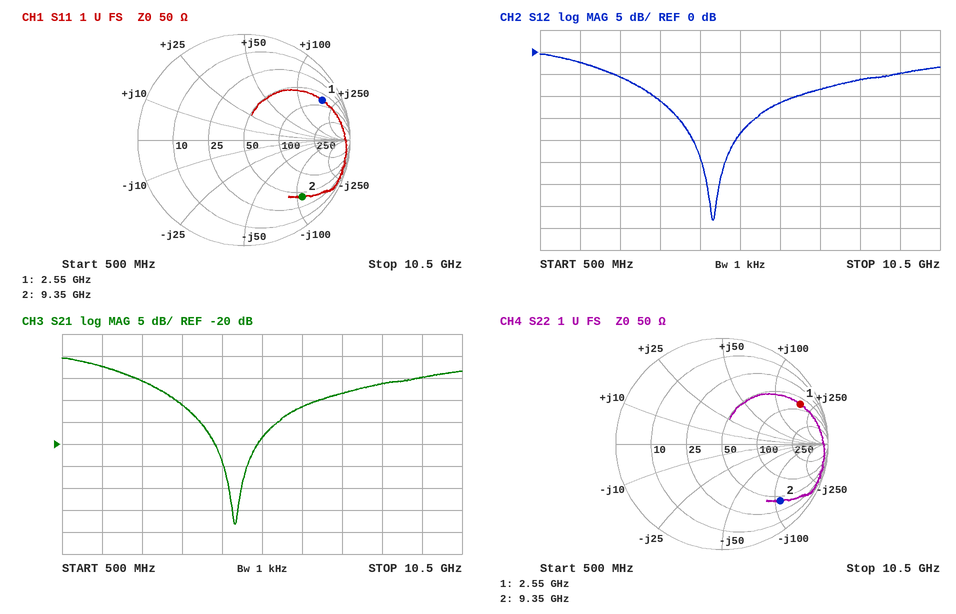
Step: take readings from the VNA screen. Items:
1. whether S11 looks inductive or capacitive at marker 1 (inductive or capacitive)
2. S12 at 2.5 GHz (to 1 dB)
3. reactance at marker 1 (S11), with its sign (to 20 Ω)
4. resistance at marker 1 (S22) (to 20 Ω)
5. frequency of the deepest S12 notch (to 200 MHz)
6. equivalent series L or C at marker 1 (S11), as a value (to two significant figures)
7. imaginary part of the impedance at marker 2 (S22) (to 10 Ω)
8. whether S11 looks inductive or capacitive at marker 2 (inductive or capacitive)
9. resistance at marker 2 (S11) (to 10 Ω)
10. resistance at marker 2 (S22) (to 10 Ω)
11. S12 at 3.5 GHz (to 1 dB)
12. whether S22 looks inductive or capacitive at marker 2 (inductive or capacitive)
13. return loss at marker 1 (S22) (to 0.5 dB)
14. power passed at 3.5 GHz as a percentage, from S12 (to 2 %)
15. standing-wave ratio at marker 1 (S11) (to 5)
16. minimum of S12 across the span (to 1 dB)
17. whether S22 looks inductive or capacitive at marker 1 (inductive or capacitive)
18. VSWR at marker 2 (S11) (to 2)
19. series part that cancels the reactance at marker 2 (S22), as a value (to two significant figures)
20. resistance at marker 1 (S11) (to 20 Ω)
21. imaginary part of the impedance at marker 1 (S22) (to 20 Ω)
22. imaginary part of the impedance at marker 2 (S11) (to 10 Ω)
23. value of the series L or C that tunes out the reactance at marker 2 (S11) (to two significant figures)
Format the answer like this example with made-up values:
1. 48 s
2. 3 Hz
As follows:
1. inductive
2. -6 dB
3. +180 Ω
4. 80 Ω
5. 4.8 GHz
6. 11 nH
7. -110 Ω
8. capacitive
9. 40 Ω
10. 40 Ω
11. -11 dB
12. capacitive
13. 1.5 dB
14. 8 %
15. 10
16. -38 dB
17. inductive
18. 8
19. 1.9 nH
20. 80 Ω
21. +180 Ω
22. -110 Ω
23. 1.9 nH
